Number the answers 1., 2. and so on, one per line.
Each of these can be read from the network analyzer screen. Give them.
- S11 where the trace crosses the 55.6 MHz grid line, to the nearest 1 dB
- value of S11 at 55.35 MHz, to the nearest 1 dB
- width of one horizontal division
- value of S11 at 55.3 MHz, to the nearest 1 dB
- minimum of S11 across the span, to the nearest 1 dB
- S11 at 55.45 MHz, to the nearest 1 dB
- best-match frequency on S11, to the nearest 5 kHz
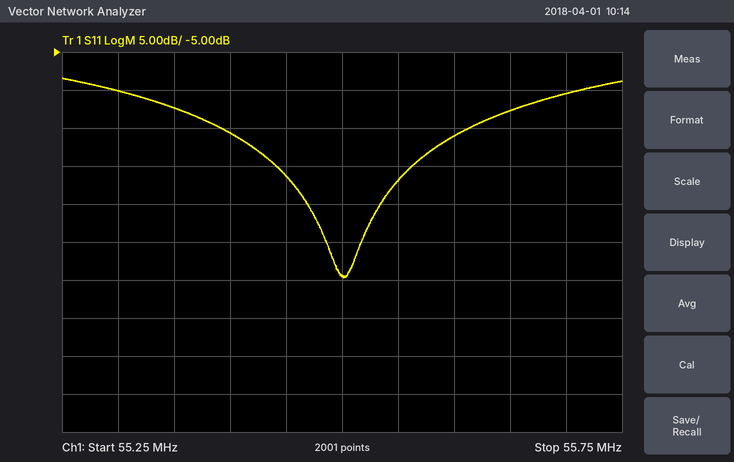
1. -16 dB
2. -12 dB
3. 50 kHz
4. -10 dB
5. -35 dB
6. -21 dB
7. 55.500 MHz
